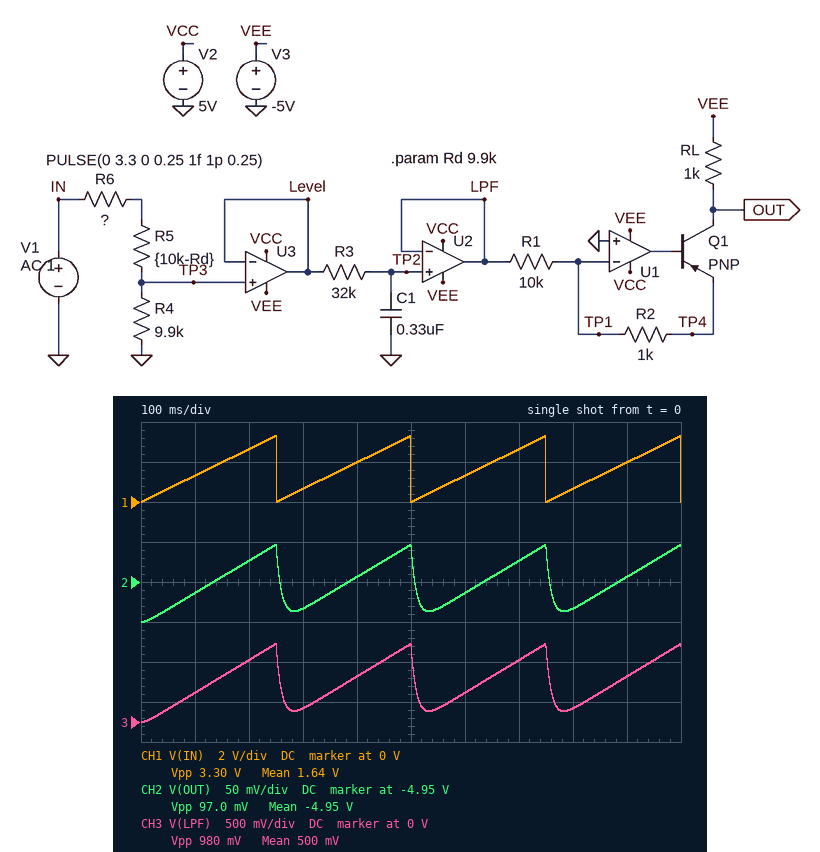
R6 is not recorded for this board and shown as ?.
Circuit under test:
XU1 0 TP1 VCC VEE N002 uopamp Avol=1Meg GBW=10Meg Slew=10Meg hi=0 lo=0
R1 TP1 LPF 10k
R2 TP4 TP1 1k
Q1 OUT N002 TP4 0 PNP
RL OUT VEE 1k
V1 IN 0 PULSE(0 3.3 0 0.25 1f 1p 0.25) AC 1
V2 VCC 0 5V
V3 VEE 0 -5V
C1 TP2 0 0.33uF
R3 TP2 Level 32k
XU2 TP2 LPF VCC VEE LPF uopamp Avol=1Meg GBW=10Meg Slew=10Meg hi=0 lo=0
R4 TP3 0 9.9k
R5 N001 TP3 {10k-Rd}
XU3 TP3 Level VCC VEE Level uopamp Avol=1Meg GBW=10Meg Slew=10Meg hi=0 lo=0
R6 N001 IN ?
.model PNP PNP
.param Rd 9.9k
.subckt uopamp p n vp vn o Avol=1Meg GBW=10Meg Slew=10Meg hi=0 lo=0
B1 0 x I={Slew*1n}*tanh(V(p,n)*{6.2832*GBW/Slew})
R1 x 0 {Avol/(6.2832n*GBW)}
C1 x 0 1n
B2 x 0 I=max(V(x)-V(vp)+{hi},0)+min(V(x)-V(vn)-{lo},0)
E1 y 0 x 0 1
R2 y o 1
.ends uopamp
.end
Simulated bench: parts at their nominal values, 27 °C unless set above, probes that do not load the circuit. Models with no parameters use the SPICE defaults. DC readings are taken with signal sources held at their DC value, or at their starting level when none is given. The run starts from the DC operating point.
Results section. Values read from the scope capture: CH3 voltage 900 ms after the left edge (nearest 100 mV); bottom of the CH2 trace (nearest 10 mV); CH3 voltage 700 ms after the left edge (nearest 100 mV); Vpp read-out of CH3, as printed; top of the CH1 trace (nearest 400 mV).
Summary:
600 mV
-5.00 V
800 mV
980 mV
3.2 V
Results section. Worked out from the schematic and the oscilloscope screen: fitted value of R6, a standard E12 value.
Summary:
22 kΩ
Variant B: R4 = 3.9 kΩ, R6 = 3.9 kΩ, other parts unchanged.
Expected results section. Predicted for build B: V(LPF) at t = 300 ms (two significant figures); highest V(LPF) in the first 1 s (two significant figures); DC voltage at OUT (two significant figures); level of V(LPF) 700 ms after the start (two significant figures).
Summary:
270 mV
1.6 V
-5.0 V
1.2 V
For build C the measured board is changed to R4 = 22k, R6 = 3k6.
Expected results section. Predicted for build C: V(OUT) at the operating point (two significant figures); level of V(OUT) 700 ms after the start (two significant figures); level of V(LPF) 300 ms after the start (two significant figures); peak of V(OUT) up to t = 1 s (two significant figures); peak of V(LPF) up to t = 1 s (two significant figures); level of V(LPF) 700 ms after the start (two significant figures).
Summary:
-5.0 V
-4.8 V
470 mV
-4.7 V
2.7 V
2.1 V
